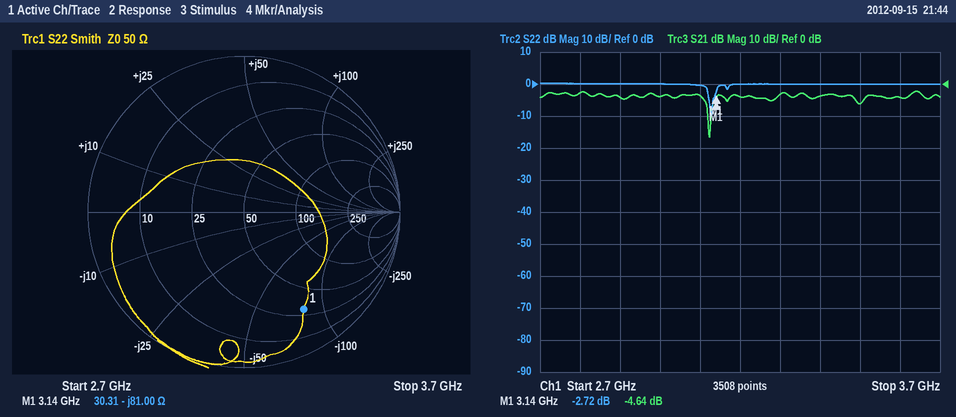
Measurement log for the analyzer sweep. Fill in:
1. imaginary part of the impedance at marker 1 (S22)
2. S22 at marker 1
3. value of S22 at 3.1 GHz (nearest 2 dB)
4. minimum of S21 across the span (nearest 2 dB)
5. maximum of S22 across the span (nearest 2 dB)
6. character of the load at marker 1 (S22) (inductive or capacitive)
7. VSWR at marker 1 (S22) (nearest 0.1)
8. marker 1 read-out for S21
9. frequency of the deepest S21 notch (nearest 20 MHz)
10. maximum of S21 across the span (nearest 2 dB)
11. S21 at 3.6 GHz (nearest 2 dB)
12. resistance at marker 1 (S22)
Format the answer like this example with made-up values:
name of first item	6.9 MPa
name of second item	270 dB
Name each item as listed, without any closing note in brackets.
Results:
imaginary part of the impedance at marker 1	-81.00 Ω
S22 at marker 1	-2.72 dB
value of S22 at 3.1 GHz	0 dB
minimum of S21 across the span	-16 dB
maximum of S22 across the span	0 dB
character of the load at marker 1 (S22)	capacitive
VSWR at marker 1 (S22)	6.4
marker 1 read-out for S21	-4.64 dB
frequency of the deepest S21 notch	3.12 GHz
maximum of S21 across the span	-2 dB
S21 at 3.6 GHz	-4 dB
resistance at marker 1	30.31 Ω
